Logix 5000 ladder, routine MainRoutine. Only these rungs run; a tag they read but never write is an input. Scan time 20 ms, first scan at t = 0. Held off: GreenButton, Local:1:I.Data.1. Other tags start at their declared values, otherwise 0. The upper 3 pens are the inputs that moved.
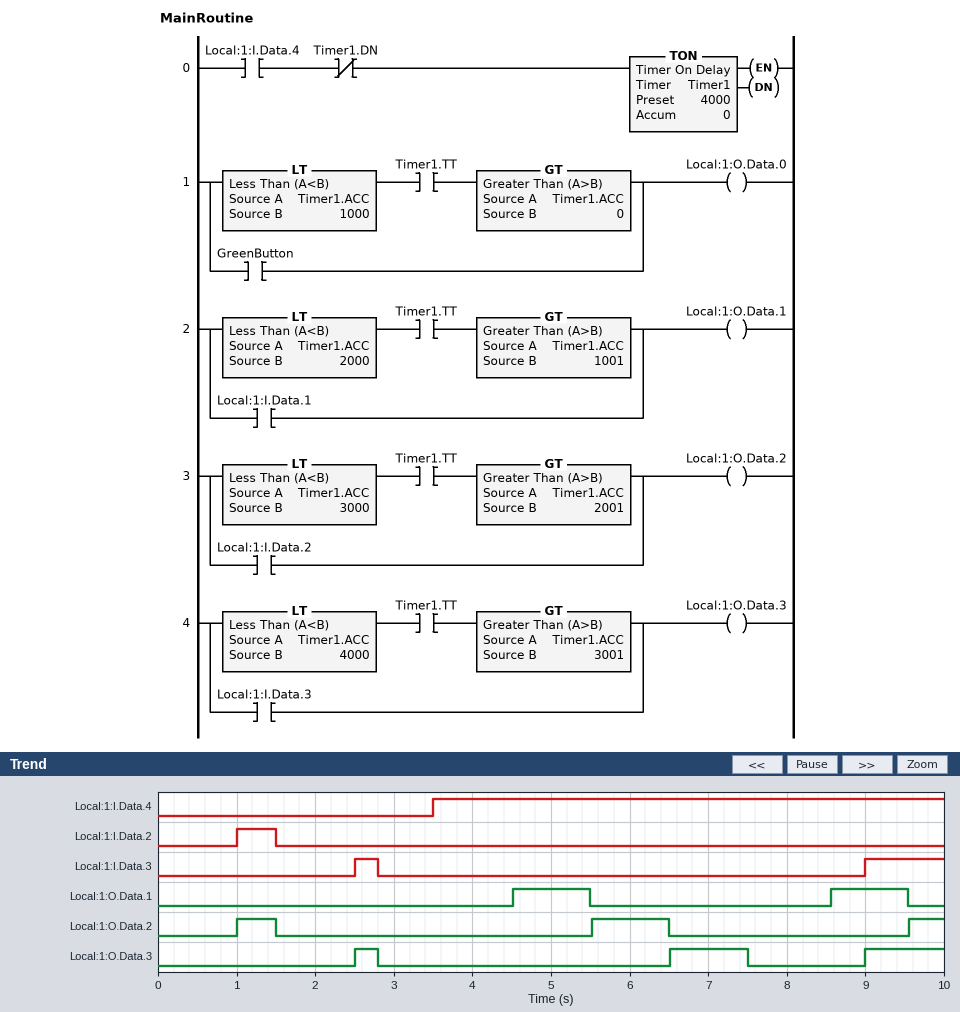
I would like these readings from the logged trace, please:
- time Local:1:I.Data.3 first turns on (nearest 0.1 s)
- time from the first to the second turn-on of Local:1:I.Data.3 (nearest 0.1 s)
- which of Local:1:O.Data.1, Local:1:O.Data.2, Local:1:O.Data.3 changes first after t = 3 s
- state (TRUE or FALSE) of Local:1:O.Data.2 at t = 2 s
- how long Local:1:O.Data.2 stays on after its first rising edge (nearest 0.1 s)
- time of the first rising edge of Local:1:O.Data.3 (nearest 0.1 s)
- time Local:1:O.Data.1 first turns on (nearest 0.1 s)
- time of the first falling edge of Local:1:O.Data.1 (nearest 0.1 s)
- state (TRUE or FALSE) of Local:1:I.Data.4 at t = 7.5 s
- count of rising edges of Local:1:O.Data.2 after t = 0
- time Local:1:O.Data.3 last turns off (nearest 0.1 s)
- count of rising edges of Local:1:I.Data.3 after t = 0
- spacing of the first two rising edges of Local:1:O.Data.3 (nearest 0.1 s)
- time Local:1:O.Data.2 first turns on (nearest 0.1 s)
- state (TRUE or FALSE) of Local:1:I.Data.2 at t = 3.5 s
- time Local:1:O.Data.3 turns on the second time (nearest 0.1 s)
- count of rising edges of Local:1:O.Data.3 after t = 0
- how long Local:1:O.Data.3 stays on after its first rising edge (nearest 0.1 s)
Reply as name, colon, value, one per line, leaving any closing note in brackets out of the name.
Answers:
time Local:1:I.Data.3 first turns on: 2.5 s
time from the first to the second turn-on of Local:1:I.Data.3: 6.5 s
which of Local:1:O.Data.1, Local:1:O.Data.2, Local:1:O.Data.3 changes first after t = 3 s: Local:1:O.Data.1
state (TRUE or FALSE) of Local:1:O.Data.2 at t = 2 s: FALSE
how long Local:1:O.Data.2 stays on after its first rising edge: 0.5 s
time of the first rising edge of Local:1:O.Data.3: 2.5 s
time Local:1:O.Data.1 first turns on: 4.5 s
time of the first falling edge of Local:1:O.Data.1: 5.5 s
state (TRUE or FALSE) of Local:1:I.Data.4 at t = 7.5 s: TRUE
count of rising edges of Local:1:O.Data.2 after t = 0: 3
time Local:1:O.Data.3 last turns off: 7.5 s
count of rising edges of Local:1:I.Data.3 after t = 0: 2
spacing of the first two rising edges of Local:1:O.Data.3: 4.0 s
time Local:1:O.Data.2 first turns on: 1.0 s
state (TRUE or FALSE) of Local:1:I.Data.2 at t = 3.5 s: FALSE
time Local:1:O.Data.3 turns on the second time: 6.5 s
count of rising edges of Local:1:O.Data.3 after t = 0: 3
how long Local:1:O.Data.3 stays on after its first rising edge: 0.3 s
